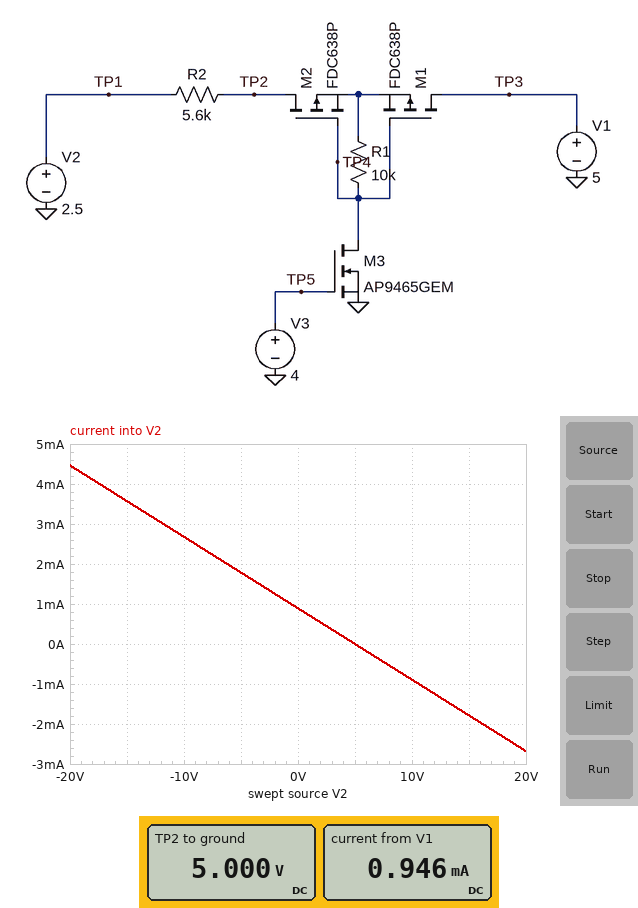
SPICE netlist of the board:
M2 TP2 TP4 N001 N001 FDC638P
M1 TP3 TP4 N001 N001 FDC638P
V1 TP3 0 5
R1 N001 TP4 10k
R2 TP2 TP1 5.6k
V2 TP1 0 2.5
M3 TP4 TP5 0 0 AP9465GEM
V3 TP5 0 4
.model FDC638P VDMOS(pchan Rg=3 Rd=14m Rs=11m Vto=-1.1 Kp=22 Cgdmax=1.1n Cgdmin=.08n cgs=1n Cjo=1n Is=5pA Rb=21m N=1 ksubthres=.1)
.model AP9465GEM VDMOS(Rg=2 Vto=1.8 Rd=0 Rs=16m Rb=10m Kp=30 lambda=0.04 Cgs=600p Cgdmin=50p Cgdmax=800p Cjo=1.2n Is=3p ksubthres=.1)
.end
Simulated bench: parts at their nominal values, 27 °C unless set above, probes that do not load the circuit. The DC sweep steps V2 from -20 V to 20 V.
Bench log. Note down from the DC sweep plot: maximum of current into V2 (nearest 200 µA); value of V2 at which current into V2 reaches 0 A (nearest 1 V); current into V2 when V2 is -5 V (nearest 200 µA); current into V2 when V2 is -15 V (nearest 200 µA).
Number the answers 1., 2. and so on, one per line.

1. 4.4 mA
2. 5 V
3. 1.8 mA
4. 3.6 mA
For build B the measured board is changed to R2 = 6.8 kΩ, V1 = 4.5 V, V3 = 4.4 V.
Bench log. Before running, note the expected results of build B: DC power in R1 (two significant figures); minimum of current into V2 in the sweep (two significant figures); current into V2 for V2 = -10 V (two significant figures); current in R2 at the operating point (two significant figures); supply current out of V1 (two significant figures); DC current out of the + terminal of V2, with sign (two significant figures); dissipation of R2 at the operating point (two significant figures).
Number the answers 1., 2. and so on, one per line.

1. 2.0 mW
2. -2.3 mA
3. 2.1 mA
4. 290 µA
5. 740 µA
6. -290 µA
7. 590 µW
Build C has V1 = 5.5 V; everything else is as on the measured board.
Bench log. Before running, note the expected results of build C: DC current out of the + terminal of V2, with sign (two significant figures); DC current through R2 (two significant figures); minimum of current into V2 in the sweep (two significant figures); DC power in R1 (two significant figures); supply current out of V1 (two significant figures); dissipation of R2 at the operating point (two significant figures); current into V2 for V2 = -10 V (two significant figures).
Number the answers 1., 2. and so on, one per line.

1. -540 µA
2. 540 µA
3. -2.6 mA
4. 3.0 mW
5. 1.1 mA
6. 1.6 mW
7. 2.8 mA
